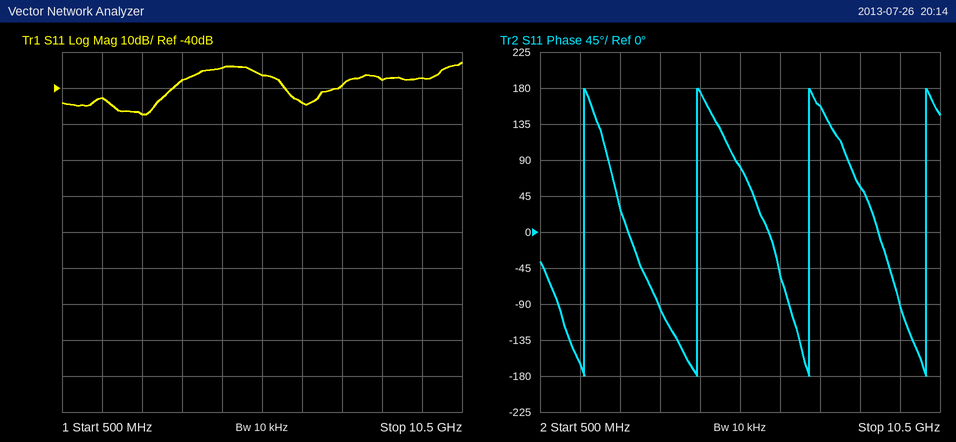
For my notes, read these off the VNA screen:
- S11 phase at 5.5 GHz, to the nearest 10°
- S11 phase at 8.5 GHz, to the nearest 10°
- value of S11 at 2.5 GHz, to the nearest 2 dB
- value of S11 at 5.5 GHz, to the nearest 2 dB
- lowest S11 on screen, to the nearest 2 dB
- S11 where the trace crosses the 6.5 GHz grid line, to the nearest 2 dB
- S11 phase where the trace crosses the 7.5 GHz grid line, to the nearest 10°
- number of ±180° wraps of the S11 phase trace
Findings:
80°
60°
-48 dB
-36 dB
-48 dB
-44 dB
160°
4
